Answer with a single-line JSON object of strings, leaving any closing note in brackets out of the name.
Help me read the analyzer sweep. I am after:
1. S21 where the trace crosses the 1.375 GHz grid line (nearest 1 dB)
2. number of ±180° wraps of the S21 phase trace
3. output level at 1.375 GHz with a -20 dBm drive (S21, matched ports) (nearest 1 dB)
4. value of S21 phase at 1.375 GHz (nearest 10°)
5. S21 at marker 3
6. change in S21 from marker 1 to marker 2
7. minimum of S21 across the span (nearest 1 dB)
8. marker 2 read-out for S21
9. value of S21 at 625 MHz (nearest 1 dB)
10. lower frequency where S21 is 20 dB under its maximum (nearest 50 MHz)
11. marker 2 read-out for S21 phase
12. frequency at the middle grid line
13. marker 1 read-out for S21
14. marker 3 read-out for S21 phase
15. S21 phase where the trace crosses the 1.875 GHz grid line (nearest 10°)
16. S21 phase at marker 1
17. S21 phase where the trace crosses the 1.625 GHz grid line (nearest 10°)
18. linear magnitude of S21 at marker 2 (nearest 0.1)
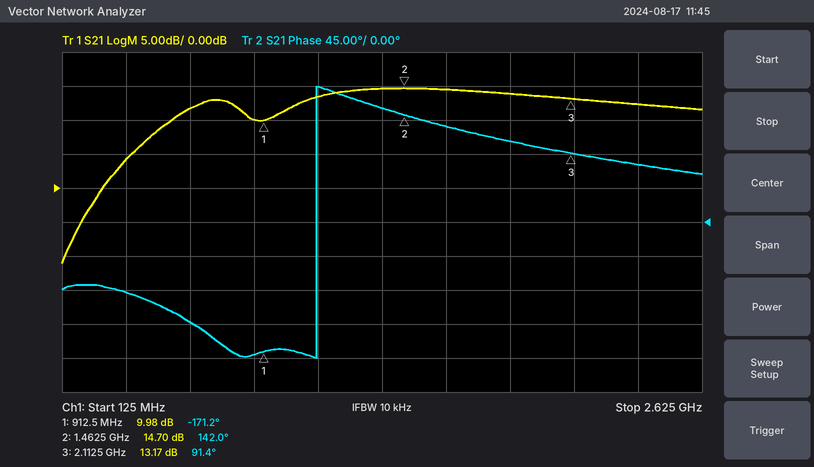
{"S21 where the trace crosses the 1.375 GHz grid line": "15 dB", "number of ±180° wraps of the S21 phase trace": "1", "output level at 1.375 GHz with a -20 dBm drive (S21, matched ports)": "-5 dBm", "value of S21 phase at 1.375 GHz": "150°", "S21 at marker 3": "13.17 dB", "change in S21 from marker 1 to marker 2": "4.72 dB", "minimum of S21 across the span": "-11 dB", "marker 2 read-out for S21": "14.70 dB", "value of S21 at 625 MHz": "12 dB", "lower frequency where S21 is 20 dB under its maximum": "200 MHz", "marker 2 read-out for S21 phase": "142.0°", "frequency at the middle grid line": "1.375 GHz", "marker 1 read-out for S21": "9.98 dB", "marker 3 read-out for S21 phase": "91.4°", "S21 phase where the trace crosses the 1.875 GHz grid line": "110°", "S21 phase at marker 1": "-171.2°", "S21 phase where the trace crosses the 1.625 GHz grid line": "130°", "linear magnitude of S21 at marker 2": "5.4"}
